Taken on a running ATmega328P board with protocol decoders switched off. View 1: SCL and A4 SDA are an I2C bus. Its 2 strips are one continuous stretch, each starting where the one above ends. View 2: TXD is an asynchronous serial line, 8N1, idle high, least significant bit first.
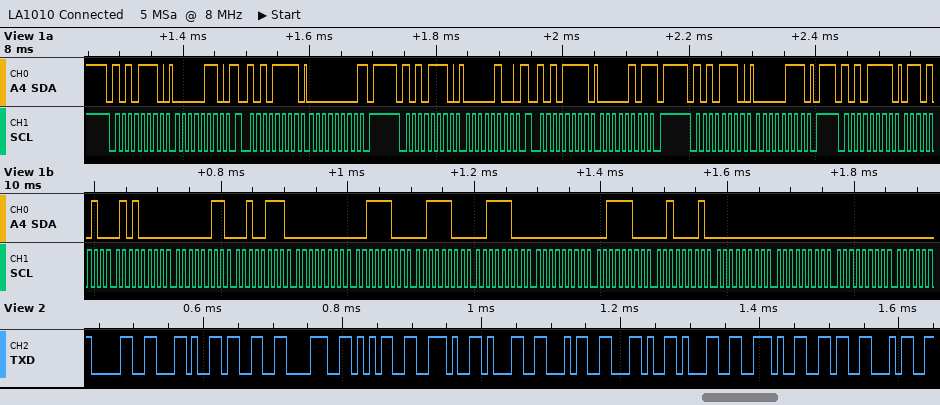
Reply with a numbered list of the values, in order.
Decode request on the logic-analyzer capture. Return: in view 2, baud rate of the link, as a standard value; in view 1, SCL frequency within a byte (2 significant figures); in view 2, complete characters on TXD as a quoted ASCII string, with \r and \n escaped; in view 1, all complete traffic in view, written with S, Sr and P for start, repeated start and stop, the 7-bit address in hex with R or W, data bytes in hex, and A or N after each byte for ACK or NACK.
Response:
1. 115200 baud
2. 100 kHz
3. "0,385.14,1.64"
4. S 57W A 06 A Sr 57R A 00 N P S 57W A 04 A Sr 57R A 05 N P S 57W A 07 A P S 57R A 6A A 50 A 03 A 27 A 00 A 3C A 3C A 3C A 00 A 3C A 21 A 00 A 00 A 00 A
